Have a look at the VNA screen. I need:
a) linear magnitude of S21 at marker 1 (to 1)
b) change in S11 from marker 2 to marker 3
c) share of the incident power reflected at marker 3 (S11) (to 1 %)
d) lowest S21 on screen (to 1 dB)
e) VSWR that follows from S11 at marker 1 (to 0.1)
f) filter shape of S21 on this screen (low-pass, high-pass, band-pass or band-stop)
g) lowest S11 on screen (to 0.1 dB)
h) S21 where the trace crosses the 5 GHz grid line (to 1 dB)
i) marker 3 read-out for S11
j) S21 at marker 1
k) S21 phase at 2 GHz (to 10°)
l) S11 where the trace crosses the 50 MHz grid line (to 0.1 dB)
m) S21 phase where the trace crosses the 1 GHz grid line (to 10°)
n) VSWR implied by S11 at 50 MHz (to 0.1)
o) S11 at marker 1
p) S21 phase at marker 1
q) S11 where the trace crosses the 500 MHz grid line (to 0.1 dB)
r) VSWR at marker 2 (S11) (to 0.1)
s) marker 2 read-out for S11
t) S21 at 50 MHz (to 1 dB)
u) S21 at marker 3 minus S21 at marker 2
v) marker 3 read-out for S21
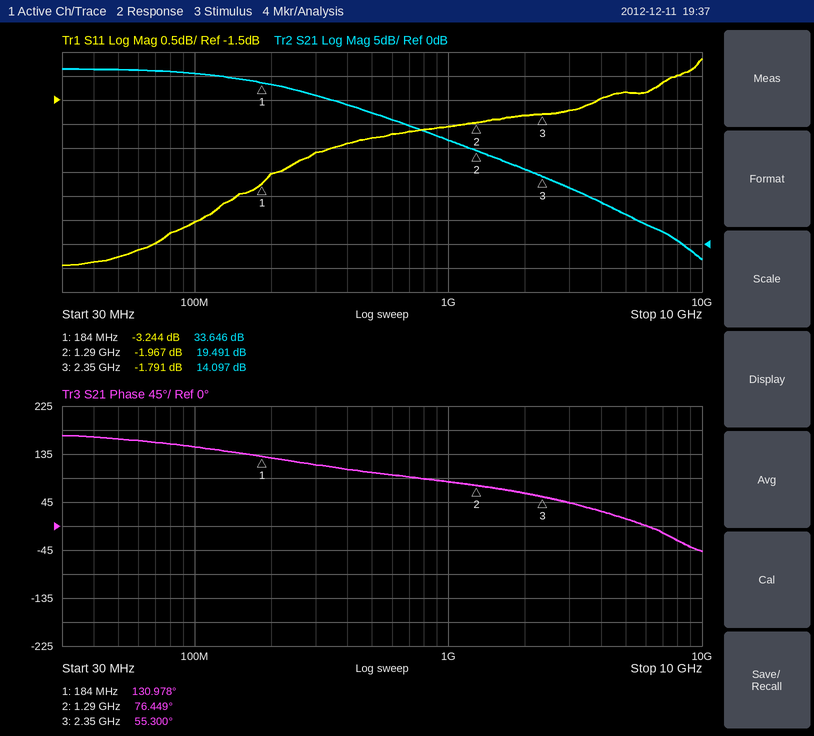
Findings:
48
0.176 dB
66 %
-3 dB
5.4
low-pass
-4.9 dB
6 dB
-1.791 dB
33.646 dB
60°
-4.8 dB
80°
3.7
-3.244 dB
130.978°
-2.3 dB
8.9
-1.967 dB
36 dB
-5.394 dB
14.097 dB
